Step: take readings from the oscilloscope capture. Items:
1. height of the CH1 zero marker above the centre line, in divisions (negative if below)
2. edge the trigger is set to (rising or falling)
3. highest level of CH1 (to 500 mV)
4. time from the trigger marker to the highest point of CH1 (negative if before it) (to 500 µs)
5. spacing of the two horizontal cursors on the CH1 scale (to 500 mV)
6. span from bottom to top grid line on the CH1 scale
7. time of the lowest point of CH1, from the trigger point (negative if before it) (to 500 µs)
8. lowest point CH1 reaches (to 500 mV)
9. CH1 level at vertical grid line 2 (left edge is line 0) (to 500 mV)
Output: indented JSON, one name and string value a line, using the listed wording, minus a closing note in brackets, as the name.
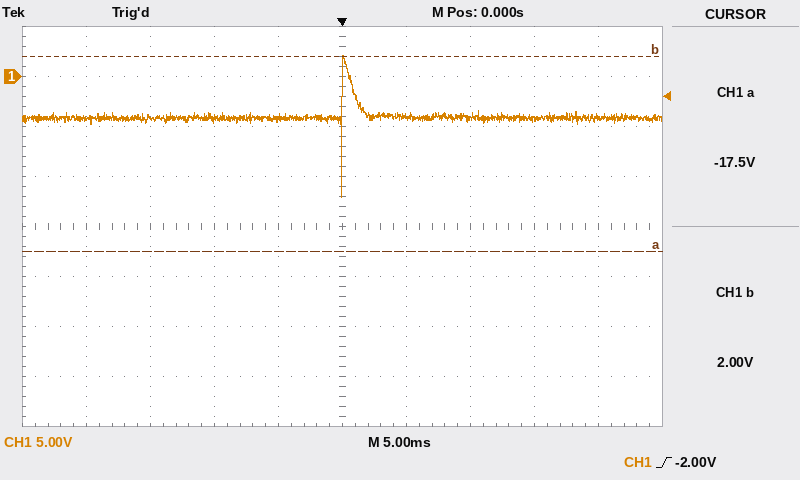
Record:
{
  "height of the CH1 zero marker above the centre line, in divisions": "+3.0 div",
  "edge the trigger is set to": "rising",
  "highest level of CH1": "2.0 V",
  "time from the trigger marker to the highest point of CH1 (negative if before it)": "0.0 ms",
  "spacing of the two horizontal cursors on the CH1 scale": "19.5 V",
  "span from bottom to top grid line on the CH1 scale": "40 V",
  "time of the lowest point of CH1, from the trigger point (negative if before it)": "0.0 ms",
  "lowest point CH1 reaches": "-12.0 V",
  "CH1 level at vertical grid line 2 (left edge is line 0)": "-4.0 V"
}
